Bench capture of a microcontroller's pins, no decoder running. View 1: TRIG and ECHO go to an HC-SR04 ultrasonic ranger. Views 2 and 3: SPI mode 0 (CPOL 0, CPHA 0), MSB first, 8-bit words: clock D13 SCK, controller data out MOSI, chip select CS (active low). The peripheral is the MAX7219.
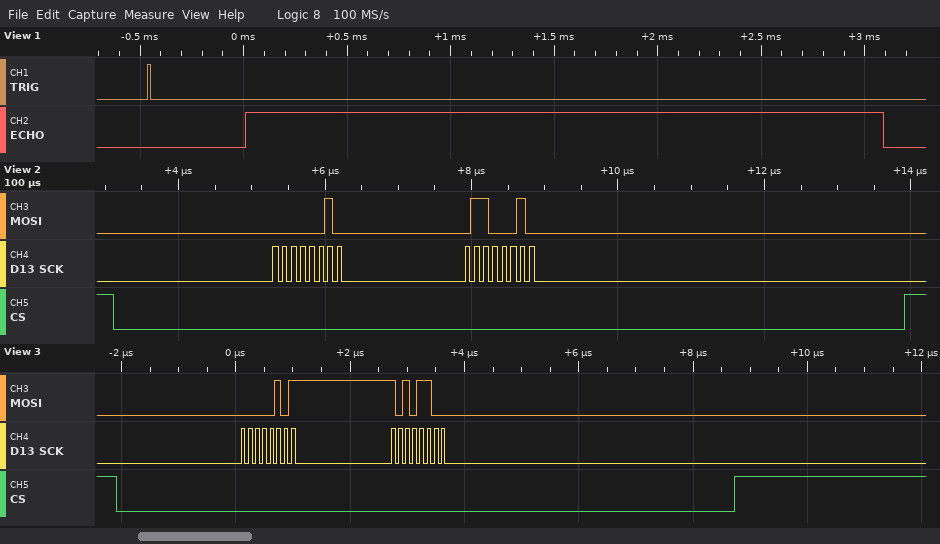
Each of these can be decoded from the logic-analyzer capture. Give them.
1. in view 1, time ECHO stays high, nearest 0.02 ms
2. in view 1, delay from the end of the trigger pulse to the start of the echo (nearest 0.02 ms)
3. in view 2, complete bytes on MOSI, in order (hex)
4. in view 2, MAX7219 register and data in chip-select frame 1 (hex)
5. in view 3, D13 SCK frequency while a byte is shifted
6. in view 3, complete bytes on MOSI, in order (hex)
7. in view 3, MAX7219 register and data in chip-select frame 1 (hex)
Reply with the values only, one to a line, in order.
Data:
3.08 ms
0.46 ms
02 62
register 0x2, data 0x62
8 MHz
05 AC
register 0x5, data 0xAC
